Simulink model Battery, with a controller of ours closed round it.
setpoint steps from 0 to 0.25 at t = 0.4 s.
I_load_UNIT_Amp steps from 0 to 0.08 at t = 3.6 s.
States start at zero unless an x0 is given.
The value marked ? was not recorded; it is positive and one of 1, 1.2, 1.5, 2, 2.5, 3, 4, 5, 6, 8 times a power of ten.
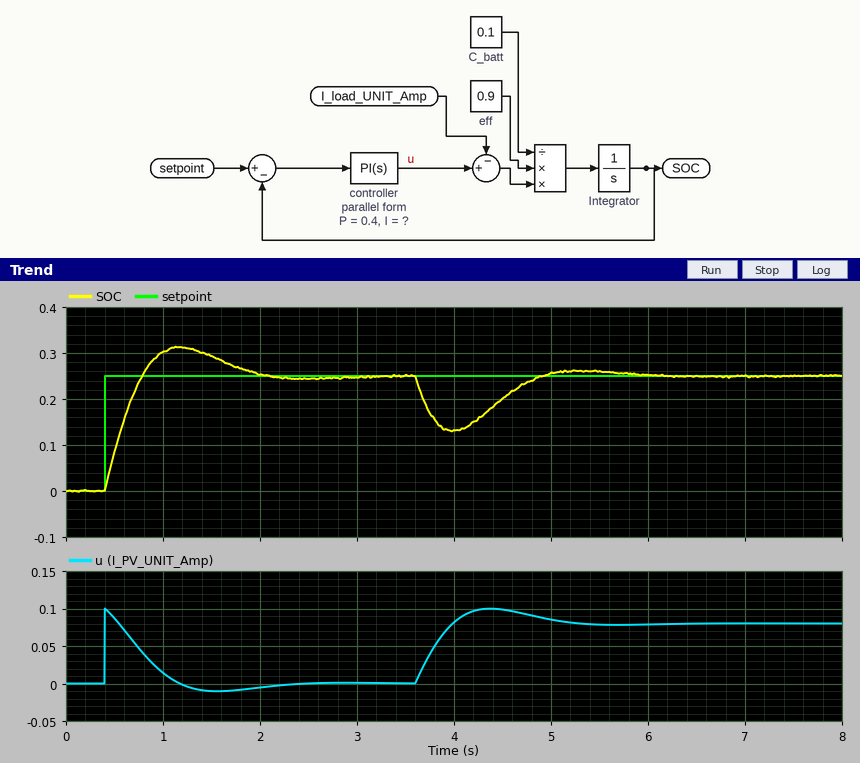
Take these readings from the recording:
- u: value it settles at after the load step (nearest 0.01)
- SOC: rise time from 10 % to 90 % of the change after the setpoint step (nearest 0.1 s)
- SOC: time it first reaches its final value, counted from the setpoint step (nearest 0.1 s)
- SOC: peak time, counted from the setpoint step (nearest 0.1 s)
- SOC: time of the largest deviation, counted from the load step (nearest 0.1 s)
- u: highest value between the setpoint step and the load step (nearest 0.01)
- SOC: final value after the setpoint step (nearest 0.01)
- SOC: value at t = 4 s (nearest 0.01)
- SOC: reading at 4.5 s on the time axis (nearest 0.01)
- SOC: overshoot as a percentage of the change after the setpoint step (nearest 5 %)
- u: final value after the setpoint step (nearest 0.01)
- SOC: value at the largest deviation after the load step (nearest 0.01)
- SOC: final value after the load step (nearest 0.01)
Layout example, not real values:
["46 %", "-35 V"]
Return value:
["0.08", "0.3 s", "0.4 s", "0.8 s", "0.4 s", "0.10", "0.25", "0.13", "0.20", "25 %", "0.00", "0.13", "0.25"]
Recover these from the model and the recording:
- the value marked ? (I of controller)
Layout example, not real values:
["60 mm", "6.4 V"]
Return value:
["1"]
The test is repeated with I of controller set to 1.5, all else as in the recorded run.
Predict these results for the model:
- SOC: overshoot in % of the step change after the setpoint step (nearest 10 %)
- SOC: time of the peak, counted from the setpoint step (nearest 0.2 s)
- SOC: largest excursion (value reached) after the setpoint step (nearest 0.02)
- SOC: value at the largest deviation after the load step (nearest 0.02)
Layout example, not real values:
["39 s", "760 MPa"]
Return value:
["30 %", "0.6 s", "0.32", "0.14"]
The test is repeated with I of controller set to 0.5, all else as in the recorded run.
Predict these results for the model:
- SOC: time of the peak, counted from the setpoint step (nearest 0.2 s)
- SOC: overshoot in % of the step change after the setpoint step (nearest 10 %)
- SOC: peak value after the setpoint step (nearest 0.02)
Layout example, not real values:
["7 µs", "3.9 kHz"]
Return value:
["1.0 s", "20 %", "0.30"]
